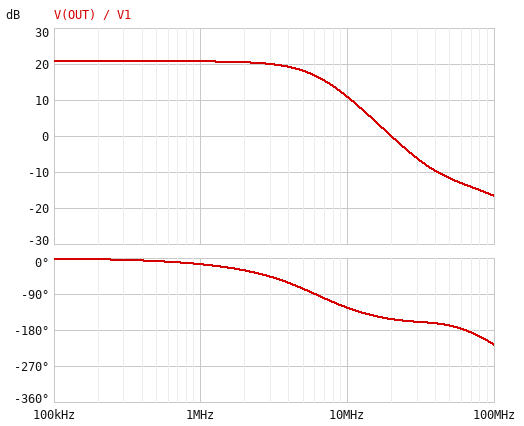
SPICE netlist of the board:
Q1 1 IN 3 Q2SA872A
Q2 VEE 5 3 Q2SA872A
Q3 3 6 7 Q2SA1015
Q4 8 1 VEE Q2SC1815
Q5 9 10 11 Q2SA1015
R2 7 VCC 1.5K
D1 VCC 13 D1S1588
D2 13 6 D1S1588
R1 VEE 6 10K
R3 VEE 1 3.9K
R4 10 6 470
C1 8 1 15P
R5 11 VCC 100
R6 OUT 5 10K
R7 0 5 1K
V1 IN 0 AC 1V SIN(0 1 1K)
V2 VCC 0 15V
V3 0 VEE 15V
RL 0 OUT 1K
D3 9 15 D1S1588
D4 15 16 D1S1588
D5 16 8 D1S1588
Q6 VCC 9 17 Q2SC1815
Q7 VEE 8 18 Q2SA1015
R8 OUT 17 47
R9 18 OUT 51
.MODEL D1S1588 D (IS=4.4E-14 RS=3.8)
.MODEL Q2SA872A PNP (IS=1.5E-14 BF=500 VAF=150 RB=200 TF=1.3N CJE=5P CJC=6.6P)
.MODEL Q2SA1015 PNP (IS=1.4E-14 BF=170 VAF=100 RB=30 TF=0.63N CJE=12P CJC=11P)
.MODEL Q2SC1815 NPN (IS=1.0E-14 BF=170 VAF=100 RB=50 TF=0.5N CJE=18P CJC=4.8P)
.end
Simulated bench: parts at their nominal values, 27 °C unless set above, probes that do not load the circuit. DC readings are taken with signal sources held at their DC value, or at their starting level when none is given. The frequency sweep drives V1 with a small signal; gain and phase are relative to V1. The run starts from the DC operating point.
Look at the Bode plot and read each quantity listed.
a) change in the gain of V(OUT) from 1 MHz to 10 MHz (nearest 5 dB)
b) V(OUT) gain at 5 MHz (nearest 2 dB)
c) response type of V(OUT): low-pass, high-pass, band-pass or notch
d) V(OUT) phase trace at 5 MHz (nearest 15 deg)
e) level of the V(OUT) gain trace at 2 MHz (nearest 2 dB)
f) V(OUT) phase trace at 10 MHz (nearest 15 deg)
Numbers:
-10 dB
18 dB
low-pass
-75 deg
20 dB
-120 deg
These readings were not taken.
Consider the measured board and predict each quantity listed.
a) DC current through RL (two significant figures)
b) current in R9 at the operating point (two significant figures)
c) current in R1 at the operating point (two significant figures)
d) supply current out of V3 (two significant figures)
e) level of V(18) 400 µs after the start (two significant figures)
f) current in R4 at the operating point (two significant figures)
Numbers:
45 µA
6.8 mA
2.9 mA
16 mA
6.2 V
31 µA
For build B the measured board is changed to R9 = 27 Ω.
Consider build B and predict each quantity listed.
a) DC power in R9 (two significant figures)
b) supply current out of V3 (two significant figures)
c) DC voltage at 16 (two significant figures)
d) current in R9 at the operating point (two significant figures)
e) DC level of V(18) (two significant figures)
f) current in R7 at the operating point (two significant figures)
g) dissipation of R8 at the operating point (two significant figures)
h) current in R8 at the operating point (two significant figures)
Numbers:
2.1 mW
18 mA
-300 mV
8.8 mA
-280 mV
3.7 µA
3.6 mW
8.7 mA
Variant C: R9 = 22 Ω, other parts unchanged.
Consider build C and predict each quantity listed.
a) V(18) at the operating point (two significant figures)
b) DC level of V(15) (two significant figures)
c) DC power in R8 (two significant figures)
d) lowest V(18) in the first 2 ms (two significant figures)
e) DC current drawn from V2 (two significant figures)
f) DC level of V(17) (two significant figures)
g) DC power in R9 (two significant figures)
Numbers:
-250 mV
420 mV
4.1 mW
-11 V
19 mA
390 mV
1.9 mW
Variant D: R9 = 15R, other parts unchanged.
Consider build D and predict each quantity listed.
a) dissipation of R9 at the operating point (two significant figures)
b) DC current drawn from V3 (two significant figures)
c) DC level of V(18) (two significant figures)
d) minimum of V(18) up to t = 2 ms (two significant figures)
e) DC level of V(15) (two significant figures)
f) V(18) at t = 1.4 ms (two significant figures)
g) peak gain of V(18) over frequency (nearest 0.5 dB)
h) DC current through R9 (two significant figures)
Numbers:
1.6 mW
20 mA
-200 mV
-11 V
470 mV
6.3 V
21.0 dB
10 mA
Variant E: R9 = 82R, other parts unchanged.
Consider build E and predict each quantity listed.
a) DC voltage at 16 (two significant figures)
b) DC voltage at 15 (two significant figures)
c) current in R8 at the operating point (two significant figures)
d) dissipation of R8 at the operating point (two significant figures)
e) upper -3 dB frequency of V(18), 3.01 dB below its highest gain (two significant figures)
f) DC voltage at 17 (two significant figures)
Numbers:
-480 mV
210 mV
5.2 mA
1.3 mW
5.2 MHz
200 mV
